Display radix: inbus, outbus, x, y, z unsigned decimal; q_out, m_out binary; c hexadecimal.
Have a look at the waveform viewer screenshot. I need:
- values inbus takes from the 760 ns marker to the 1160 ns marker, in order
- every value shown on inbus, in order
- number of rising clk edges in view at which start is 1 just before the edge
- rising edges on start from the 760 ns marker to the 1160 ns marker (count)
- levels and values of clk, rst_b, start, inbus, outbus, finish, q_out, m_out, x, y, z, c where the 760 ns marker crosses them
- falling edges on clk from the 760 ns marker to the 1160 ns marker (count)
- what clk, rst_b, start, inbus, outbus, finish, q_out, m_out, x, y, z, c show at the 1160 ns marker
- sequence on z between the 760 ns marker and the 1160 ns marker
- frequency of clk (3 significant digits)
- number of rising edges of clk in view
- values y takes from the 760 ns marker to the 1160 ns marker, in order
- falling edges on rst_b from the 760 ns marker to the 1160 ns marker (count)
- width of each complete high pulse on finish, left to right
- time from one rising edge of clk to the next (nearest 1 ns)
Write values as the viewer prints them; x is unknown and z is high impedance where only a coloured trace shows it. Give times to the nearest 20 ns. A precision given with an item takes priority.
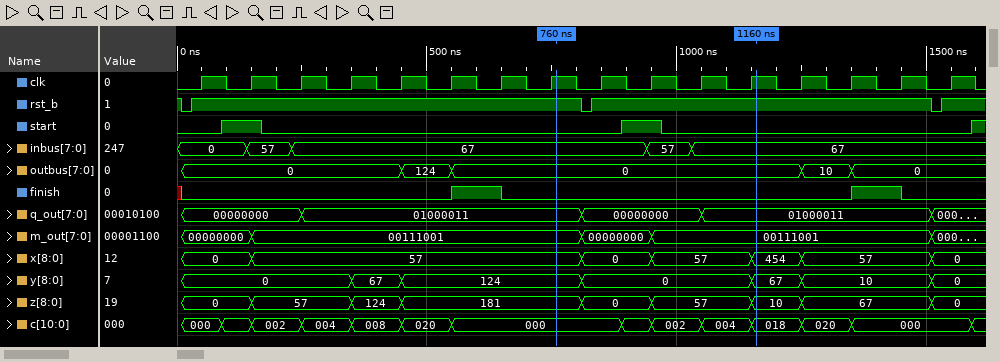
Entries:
67, 57, 67
0, 57, 67, 57, 67
2
1
clk=1, rst_b=1, start=0, inbus=67, outbus=0, finish=0, q_out=01000011, m_out=00111001, x=57, y=124, z=181, c=000
4
clk=1, rst_b=1, start=0, inbus=67, outbus=0, finish=0, q_out=01000011, m_out=00111001, x=454, y=67, z=10, c=018
181, 0, 57, 10
10.0 MHz
16
124, 0, 67
1
100 ns, 100 ns
100 ns
